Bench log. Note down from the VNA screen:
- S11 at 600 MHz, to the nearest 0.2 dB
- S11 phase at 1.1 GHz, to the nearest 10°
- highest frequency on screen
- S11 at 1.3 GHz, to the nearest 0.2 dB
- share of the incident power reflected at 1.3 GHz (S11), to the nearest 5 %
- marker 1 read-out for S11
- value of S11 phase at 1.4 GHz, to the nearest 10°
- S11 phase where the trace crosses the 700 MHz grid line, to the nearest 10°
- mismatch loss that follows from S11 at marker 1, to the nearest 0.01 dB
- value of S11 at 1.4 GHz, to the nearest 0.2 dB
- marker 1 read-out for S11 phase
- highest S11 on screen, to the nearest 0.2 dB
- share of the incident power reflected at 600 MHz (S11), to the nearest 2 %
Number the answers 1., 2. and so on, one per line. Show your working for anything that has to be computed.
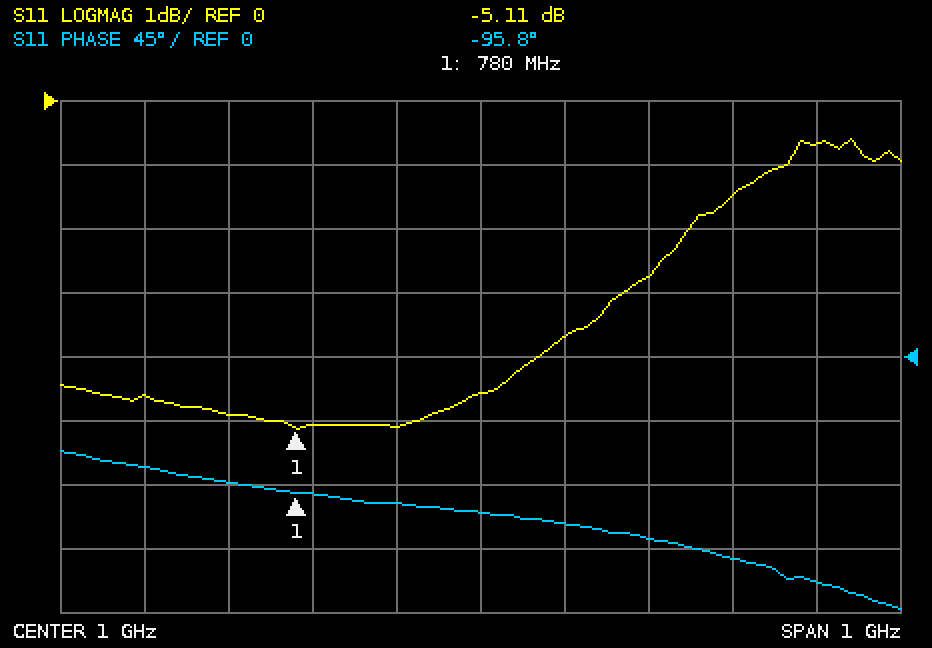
1. -4.6 dB
2. -120°
3. 1.5 GHz
4. -1.4 dB
5. 10^(-1.4/10) ≈ 72.4 %, so 70 % to the nearest 5 %
6. -5.11 dB
7. -160°
8. -90°
9. −10 log10(1 − 10^(-5.11/10)) ≈ 1.60 dB
10. -0.6 dB
11. -95.8°
12. -0.6 dB
13. 10^(-4.6/10) ≈ 34.7 %, so 34 % to the nearest 2 %
